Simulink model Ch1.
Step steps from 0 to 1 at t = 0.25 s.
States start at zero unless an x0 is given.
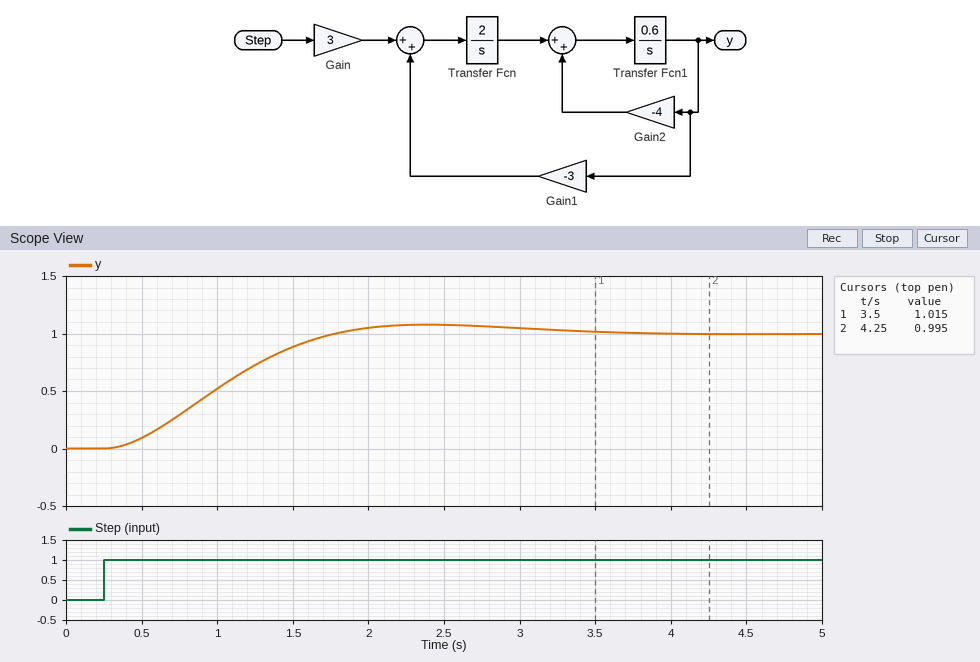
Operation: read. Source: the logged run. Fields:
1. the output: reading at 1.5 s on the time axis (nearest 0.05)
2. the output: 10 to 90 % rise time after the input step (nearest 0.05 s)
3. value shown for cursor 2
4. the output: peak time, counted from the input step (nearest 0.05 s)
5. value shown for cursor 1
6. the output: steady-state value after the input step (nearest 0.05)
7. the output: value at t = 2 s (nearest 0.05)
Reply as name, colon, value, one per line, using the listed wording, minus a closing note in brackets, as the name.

the output: reading at 1.5 s on the time axis: 0.90
the output: 10 to 90 % rise time after the input step: 1.00 s
value shown for cursor 2: 0.995
the output: peak time, counted from the input step: 2.15 s
value shown for cursor 1: 1.015
the output: steady-state value after the input step: 1.00
the output: value at t = 2 s: 1.05
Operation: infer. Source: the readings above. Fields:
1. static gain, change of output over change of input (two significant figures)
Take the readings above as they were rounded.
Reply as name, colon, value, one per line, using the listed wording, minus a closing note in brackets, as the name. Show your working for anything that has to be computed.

static gain, change of output over change of input: (1 - 0) / (1 - 0) = 1.0
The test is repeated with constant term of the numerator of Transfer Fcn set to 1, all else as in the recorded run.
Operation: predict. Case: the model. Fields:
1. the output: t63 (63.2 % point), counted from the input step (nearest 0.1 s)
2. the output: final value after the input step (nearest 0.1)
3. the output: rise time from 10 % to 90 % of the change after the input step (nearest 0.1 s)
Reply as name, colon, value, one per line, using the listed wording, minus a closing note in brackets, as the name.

the output: t63 (63.2 % point), counted from the input step: 1.5 s
the output: final value after the input step: 1.0
the output: rise time from 10 % to 90 % of the change after the input step: 2.1 s
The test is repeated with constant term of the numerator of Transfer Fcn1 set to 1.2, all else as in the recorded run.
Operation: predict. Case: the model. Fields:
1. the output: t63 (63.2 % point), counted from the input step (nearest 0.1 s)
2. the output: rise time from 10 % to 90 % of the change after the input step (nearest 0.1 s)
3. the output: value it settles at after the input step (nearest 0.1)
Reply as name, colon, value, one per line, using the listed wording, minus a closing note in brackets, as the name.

the output: t63 (63.2 % point), counted from the input step: 0.7 s
the output: rise time from 10 % to 90 % of the change after the input step: 1.1 s
the output: value it settles at after the input step: 1.0
